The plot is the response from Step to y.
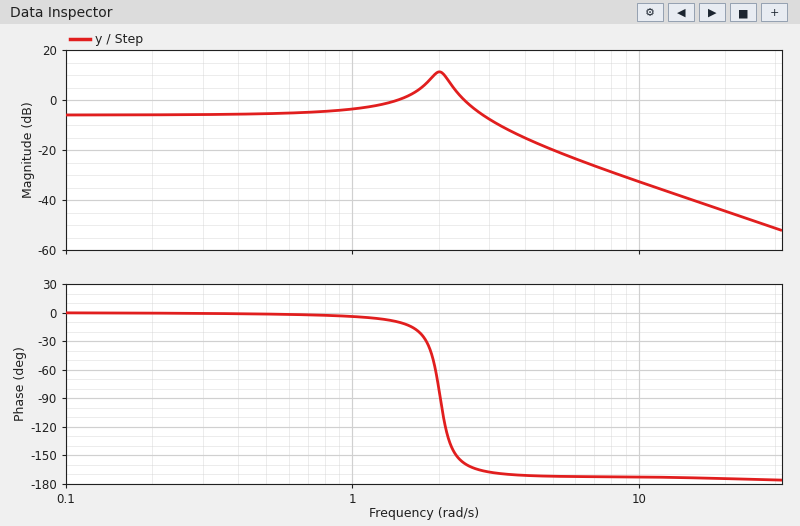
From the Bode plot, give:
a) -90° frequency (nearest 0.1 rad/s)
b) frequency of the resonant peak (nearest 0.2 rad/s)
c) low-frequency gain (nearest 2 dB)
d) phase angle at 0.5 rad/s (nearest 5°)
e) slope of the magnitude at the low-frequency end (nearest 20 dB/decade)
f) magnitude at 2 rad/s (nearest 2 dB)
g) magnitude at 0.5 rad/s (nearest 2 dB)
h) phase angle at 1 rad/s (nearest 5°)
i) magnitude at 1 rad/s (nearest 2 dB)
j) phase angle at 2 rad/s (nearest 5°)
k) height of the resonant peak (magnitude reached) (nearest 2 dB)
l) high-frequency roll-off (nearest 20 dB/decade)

2.0 rad/s
2.0 rad/s
-6 dB
0°
0 dB/decade
12 dB
-6 dB
-5°
-4 dB
-80°
12 dB
-40 dB/decade
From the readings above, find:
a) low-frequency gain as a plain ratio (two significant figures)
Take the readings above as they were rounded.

0.50
